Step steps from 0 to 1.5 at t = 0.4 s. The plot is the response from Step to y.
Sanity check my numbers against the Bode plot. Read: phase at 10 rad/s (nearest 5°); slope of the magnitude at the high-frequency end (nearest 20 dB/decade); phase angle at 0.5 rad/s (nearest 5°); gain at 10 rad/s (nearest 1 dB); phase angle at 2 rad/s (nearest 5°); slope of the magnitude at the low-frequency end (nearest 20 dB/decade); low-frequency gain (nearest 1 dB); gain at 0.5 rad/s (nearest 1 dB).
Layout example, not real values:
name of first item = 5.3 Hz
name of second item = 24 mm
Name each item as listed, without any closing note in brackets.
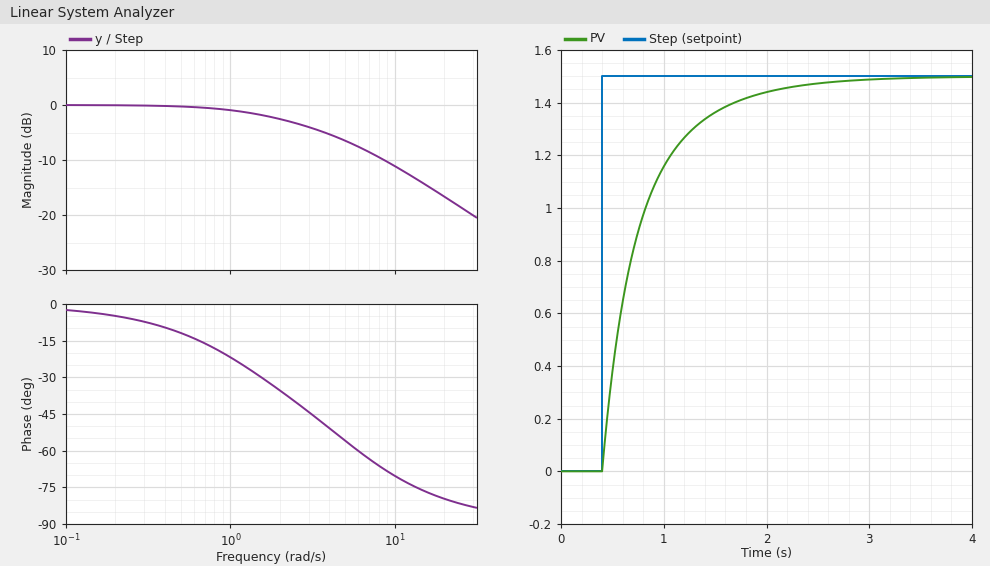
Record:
phase at 10 rad/s = -70°
slope of the magnitude at the high-frequency end = -20 dB/decade
phase angle at 0.5 rad/s = -10°
gain at 10 rad/s = -11 dB
phase angle at 2 rad/s = -35°
slope of the magnitude at the low-frequency end = 0 dB/decade
low-frequency gain = 0 dB
gain at 0.5 rad/s = 0 dB
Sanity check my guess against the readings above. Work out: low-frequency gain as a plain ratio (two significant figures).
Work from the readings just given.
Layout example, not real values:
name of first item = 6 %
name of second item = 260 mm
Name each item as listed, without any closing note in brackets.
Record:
low-frequency gain as a plain ratio = 1.0
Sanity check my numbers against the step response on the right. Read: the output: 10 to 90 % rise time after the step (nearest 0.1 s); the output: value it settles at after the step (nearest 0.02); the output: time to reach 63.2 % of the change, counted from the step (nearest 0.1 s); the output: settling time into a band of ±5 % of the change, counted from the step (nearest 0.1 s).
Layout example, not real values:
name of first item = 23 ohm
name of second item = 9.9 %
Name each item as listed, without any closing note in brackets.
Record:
the output: 10 to 90 % rise time after the step = 1.0 s
the output: value it settles at after the step = 1.50
the output: time to reach 63.2 % of the change, counted from the step = 0.4 s
the output: settling time into a band of ±5 % of the change, counted from the step = 1.5 s
